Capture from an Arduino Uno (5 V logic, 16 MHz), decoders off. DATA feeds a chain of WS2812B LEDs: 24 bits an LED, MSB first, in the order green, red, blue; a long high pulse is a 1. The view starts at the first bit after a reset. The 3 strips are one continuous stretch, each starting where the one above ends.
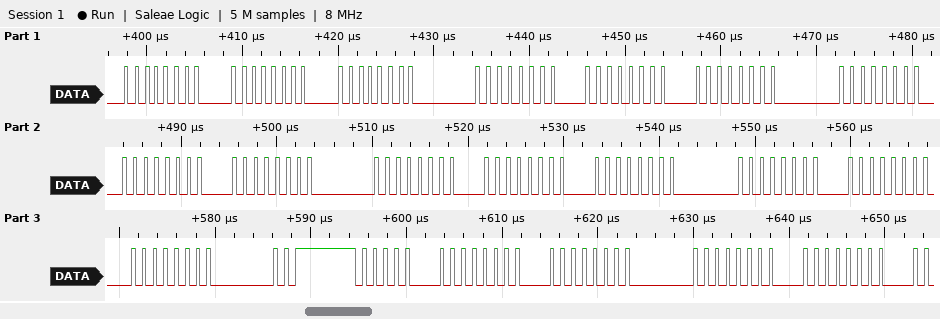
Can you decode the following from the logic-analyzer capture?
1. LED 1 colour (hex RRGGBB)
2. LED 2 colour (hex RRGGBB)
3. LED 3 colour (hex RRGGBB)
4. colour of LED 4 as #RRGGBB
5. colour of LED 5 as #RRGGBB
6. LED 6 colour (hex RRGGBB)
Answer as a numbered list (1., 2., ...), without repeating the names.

1. #000000
2. #000000
3. #000000
4. #000000
5. #000000
6. #002000
